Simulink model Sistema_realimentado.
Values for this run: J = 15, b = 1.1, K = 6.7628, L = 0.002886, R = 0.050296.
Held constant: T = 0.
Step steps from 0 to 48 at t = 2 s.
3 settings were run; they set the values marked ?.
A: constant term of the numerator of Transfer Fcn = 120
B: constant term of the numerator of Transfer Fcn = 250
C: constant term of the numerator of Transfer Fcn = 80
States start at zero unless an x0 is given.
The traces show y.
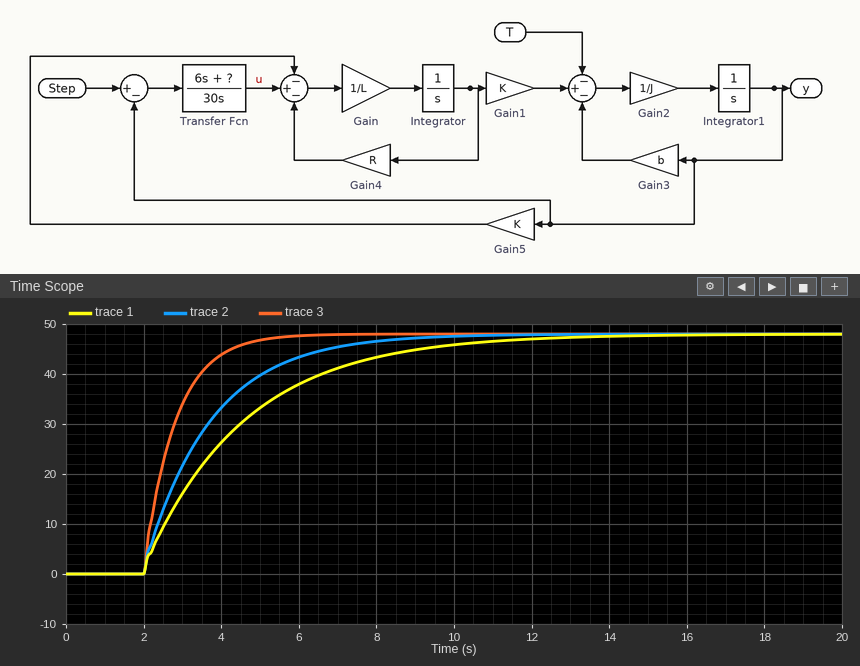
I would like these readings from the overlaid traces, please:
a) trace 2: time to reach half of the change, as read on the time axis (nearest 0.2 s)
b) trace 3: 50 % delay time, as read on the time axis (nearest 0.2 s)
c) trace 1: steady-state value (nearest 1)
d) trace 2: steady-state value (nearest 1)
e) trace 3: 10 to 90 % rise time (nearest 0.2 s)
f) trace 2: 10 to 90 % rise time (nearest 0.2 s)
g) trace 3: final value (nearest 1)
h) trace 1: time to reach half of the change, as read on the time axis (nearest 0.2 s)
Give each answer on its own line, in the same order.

3.2 s
2.6 s
48
48
1.8 s
3.8 s
48
3.8 s
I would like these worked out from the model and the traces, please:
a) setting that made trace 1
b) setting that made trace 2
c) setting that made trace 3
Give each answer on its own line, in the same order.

C
A
B
